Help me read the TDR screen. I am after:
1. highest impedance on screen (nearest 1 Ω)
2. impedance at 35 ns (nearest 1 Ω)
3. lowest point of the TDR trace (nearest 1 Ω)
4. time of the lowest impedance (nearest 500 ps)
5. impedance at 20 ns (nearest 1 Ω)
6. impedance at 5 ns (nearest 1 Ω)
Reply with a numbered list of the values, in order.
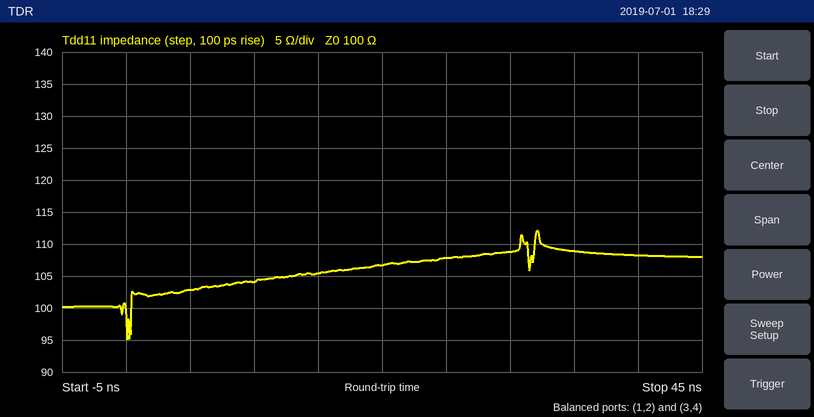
1. 112 Ω
2. 109 Ω
3. 95 Ω
4. 0.0 ns
5. 107 Ω
6. 103 Ω
